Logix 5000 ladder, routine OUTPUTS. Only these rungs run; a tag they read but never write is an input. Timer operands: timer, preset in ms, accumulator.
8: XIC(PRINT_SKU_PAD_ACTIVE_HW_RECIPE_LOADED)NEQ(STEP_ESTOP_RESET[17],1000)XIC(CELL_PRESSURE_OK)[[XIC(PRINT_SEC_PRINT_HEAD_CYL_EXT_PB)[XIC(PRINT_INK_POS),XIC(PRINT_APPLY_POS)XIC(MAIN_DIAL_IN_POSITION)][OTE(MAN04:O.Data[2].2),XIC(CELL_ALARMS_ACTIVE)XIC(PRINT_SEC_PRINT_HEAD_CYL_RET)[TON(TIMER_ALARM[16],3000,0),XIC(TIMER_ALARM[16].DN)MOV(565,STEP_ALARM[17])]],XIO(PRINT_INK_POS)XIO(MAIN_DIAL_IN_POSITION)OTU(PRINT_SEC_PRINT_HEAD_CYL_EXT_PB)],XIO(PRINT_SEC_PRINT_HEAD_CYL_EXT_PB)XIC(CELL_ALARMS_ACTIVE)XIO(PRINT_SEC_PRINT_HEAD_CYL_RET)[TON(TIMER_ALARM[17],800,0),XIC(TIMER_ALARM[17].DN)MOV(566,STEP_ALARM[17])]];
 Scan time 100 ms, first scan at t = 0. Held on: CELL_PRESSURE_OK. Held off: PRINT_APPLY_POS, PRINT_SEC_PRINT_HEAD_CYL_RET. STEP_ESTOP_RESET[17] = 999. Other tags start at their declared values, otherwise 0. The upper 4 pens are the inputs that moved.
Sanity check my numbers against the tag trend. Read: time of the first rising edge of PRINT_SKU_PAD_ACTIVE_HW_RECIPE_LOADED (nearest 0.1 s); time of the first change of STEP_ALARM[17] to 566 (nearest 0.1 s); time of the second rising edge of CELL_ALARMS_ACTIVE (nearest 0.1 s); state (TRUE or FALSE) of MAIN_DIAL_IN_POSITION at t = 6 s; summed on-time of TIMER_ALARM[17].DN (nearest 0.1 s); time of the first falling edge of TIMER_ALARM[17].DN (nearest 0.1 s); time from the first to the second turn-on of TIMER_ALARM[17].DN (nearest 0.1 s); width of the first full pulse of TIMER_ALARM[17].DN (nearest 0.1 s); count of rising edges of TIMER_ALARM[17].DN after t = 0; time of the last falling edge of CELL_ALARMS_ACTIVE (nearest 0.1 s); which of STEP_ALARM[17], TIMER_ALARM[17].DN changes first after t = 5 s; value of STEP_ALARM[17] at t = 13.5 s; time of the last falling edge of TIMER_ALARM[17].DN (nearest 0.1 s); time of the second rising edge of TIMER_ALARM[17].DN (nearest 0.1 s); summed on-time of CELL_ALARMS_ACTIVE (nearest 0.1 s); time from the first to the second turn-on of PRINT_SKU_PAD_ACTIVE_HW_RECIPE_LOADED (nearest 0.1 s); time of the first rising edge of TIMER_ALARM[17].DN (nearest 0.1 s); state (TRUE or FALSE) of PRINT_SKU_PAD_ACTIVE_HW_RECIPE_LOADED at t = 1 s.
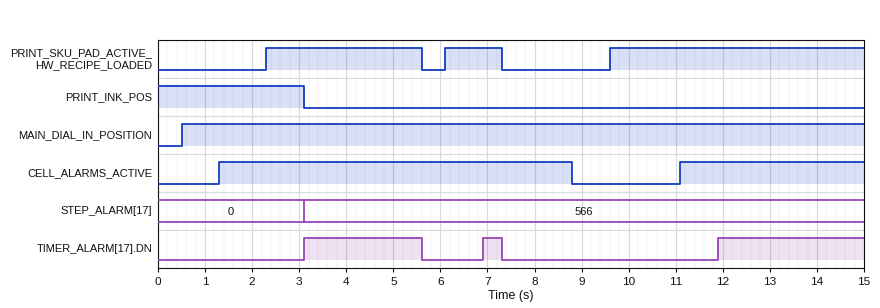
2.3 s
3.1 s
11.1 s
TRUE
6.0 s
5.6 s
3.8 s
2.5 s
3
8.8 s
TIMER_ALARM[17].DN
566
7.3 s
6.9 s
11.4 s
3.8 s
3.1 s
FALSE
